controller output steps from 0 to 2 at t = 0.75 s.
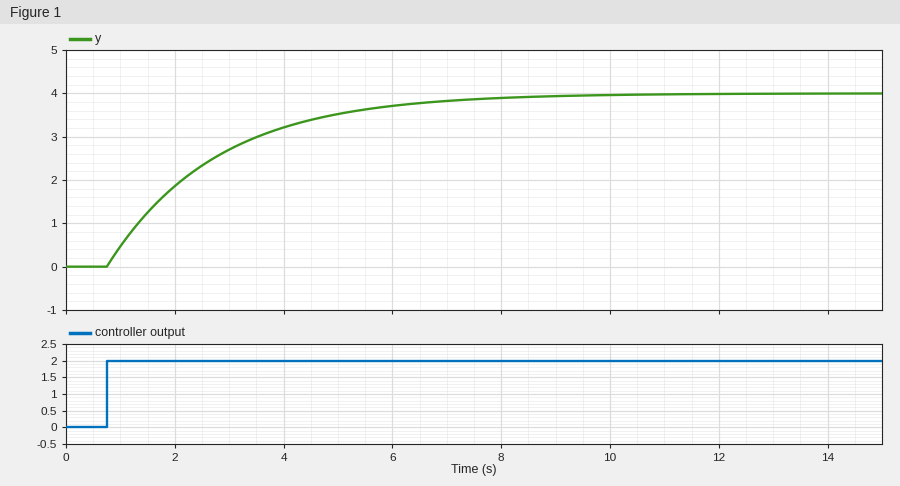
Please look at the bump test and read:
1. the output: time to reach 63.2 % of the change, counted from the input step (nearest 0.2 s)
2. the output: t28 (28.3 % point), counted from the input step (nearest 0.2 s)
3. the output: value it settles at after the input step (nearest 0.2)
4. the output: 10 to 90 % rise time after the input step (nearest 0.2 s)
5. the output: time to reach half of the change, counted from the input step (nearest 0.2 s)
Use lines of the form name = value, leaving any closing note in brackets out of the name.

the output: time to reach 63.2 % of the change, counted from the input step = 2.0 s
the output: t28 (28.3 % point), counted from the input step = 0.6 s
the output: value it settles at after the input step = 4.0
the output: 10 to 90 % rise time after the input step = 4.4 s
the output: time to reach half of the change, counted from the input step = 1.4 s
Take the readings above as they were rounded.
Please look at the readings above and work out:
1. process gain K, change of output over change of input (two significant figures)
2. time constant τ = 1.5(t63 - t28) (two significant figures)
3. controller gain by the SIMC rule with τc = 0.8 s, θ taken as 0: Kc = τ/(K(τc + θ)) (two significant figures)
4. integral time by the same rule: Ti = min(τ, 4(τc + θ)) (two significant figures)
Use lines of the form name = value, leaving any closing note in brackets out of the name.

process gain K, change of output over change of input = 2.0
time constant τ = 1.5(t63 - t28) = 2.1 s
controller gain by the SIMC rule with τc = 0.8 s, θ taken as 0: Kc = τ/(K(τc + θ)) = 1.3
integral time by the same rule: Ti = min(τ, 4(τc + θ)) = 2.1 s
